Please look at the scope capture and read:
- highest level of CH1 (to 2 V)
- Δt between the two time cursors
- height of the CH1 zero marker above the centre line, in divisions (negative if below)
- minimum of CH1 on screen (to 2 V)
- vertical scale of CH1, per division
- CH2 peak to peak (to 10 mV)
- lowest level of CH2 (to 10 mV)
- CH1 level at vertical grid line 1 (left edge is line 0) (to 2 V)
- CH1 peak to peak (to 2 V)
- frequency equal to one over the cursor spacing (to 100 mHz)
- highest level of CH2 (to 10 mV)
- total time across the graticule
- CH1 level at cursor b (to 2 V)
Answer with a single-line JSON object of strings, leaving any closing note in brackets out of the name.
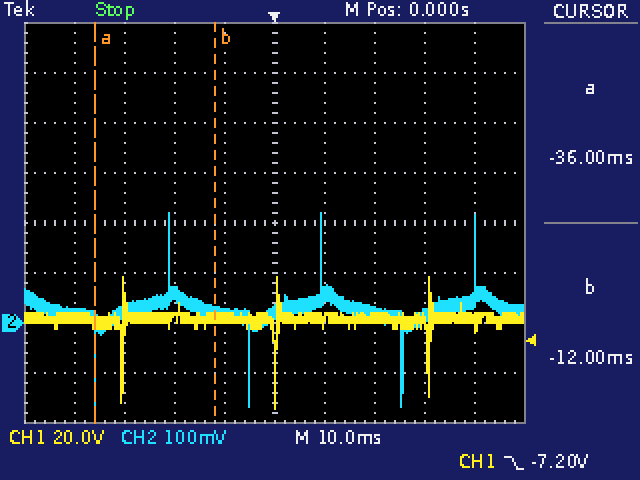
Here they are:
{"highest level of CH1": "18 V", "Δt between the two time cursors": "24 ms", "height of the CH1 zero marker above the centre line, in divisions": "-2.0 div", "minimum of CH1 on screen": "-34 V", "vertical scale of CH1, per division": "20 V", "CH2 peak to peak": "390 mV", "lowest level of CH2": "-170 mV", "CH1 level at vertical grid line 1 (left edge is line 0)": "2 V", "CH1 peak to peak": "52 V", "frequency equal to one over the cursor spacing": "41.7 Hz", "highest level of CH2": "220 mV", "total time across the graticule": "100 ms", "CH1 level at cursor b": "2 V"}
